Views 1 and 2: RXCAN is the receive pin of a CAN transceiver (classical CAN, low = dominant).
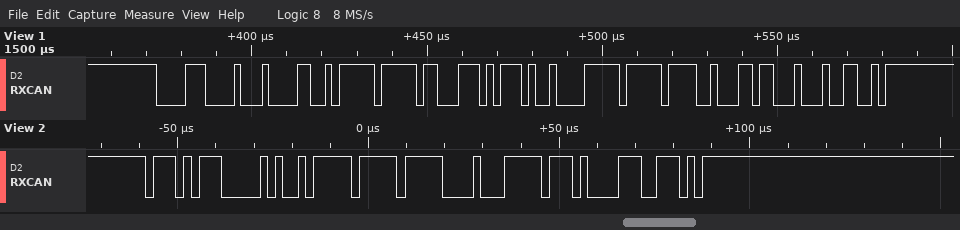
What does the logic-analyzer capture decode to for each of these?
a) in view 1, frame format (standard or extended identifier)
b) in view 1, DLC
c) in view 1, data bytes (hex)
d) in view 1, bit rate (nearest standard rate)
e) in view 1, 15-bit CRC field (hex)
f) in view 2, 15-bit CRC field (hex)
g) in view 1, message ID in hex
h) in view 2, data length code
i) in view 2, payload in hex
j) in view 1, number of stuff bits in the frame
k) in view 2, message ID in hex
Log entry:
standard
8
65 FF E3 AE 90 FF FC 8D
500 kbit/s
0x444C
0x21CE
0x0E1
4
BF FF 88 FF
4
0x75C
